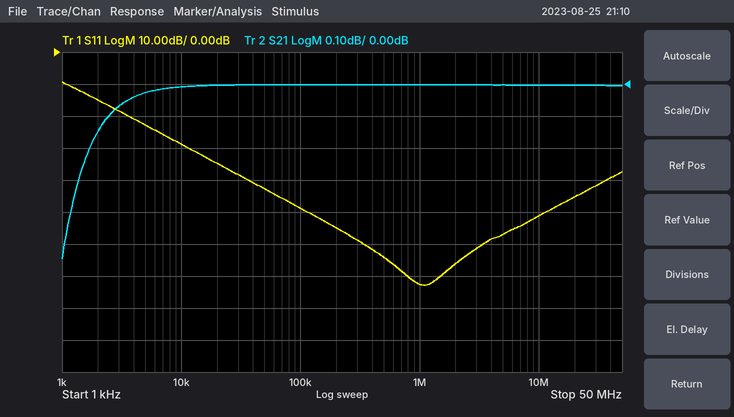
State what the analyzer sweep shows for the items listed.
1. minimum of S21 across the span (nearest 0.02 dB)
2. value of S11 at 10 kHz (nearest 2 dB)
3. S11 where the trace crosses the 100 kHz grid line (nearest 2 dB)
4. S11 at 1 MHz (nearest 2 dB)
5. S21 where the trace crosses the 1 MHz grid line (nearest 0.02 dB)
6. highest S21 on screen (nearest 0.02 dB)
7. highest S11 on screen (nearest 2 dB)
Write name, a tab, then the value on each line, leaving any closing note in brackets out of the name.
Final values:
minimum of S21 across the span	-0.54 dB
value of S11 at 10 kHz	-28 dB
S11 where the trace crosses the 100 kHz grid line	-48 dB
S11 at 1 MHz	-72 dB
S21 where the trace crosses the 1 MHz grid line	0.00 dB
highest S21 on screen	0.00 dB
highest S11 on screen	-10 dB
